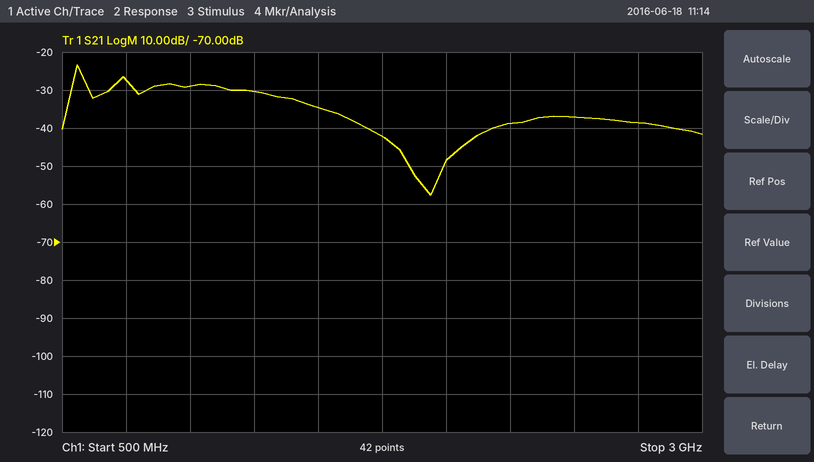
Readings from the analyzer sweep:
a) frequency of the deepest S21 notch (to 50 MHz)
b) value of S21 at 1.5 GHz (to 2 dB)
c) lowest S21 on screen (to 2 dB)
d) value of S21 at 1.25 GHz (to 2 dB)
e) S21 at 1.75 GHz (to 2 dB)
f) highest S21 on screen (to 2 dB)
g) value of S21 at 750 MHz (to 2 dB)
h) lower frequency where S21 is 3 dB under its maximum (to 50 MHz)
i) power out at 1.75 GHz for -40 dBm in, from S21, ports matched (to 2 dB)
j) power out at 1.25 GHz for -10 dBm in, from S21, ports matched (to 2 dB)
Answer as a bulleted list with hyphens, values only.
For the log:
- 1.95 GHz
- -34 dB
- -58 dB
- -30 dB
- -42 dB
- -24 dB
- -28 dB
- 550 MHz
- -82 dBm
- -40 dBm
